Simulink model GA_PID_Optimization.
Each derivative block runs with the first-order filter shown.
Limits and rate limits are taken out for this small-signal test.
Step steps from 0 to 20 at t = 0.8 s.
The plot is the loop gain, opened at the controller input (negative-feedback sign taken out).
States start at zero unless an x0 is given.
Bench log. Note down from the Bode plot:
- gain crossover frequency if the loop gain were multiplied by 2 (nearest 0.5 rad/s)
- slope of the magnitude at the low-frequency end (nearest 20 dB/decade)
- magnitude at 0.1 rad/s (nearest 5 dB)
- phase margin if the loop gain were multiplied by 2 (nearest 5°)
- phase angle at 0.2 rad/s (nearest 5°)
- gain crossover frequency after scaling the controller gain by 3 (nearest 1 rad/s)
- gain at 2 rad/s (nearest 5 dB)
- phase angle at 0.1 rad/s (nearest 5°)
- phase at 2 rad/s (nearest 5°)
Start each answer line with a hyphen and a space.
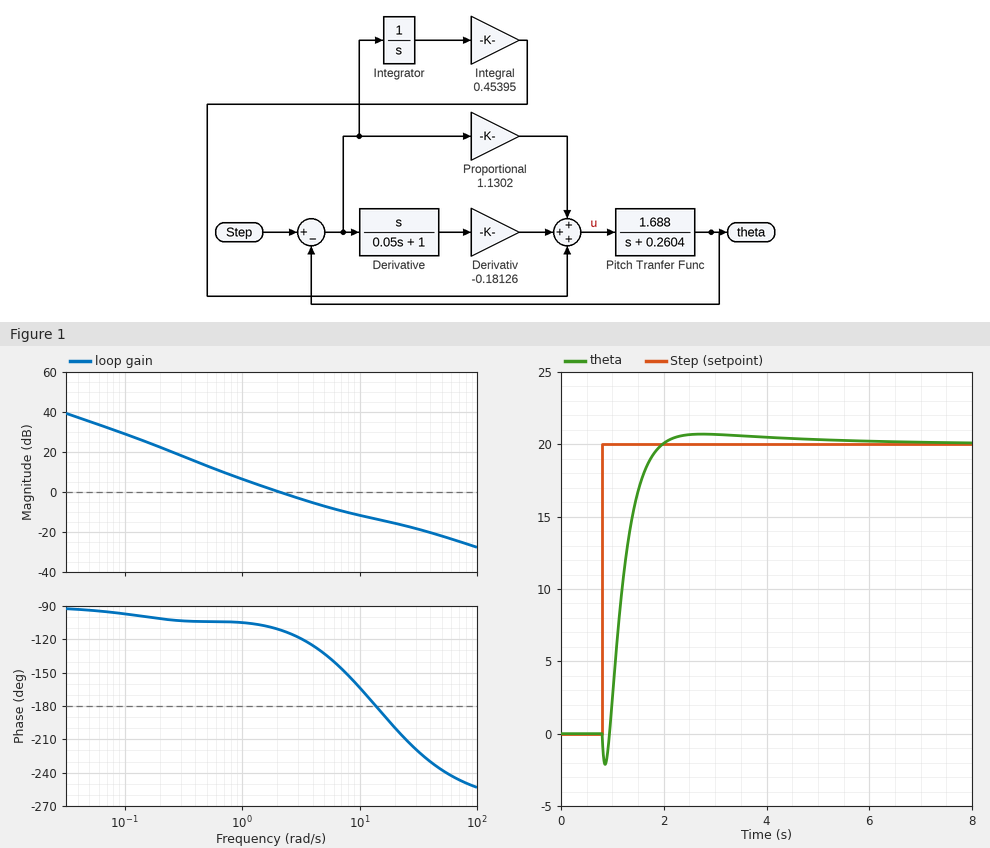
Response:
- 4.5 rad/s
- -20 dB/decade
- 30 dB
- 50°
- -100°
- 7 rad/s
- 0 dB
- -95°
- -110°
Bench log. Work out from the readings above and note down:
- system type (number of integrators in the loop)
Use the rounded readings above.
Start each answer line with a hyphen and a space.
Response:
- 1
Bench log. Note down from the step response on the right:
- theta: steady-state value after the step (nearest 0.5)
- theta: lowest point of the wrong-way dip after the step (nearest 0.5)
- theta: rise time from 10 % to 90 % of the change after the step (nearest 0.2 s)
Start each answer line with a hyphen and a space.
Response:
- 20.0
- -2.0
- 0.6 s
